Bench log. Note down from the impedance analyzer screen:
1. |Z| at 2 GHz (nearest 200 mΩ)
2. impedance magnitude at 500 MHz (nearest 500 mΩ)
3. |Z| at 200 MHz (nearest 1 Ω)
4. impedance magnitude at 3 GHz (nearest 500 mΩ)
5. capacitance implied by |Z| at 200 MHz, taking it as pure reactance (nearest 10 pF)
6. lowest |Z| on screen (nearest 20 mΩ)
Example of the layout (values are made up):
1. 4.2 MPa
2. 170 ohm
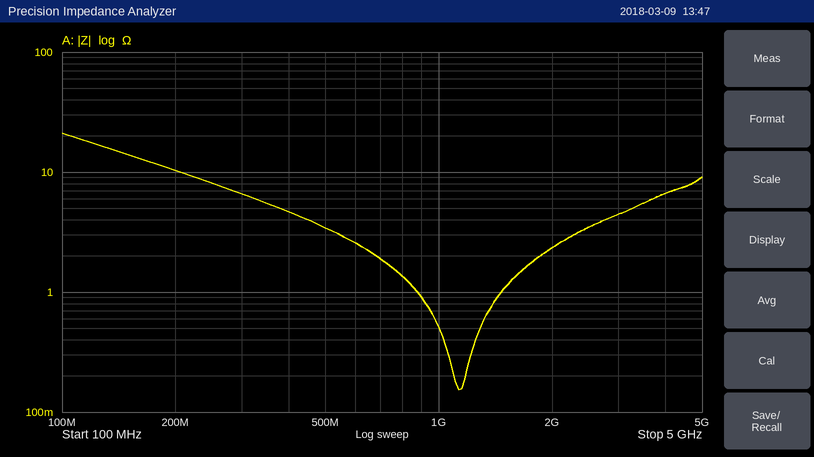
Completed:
1. 2.4 Ω
2. 3.5 Ω
3. 10 Ω
4. 4.5 Ω
5. 80 pF
6. 160 mΩ
